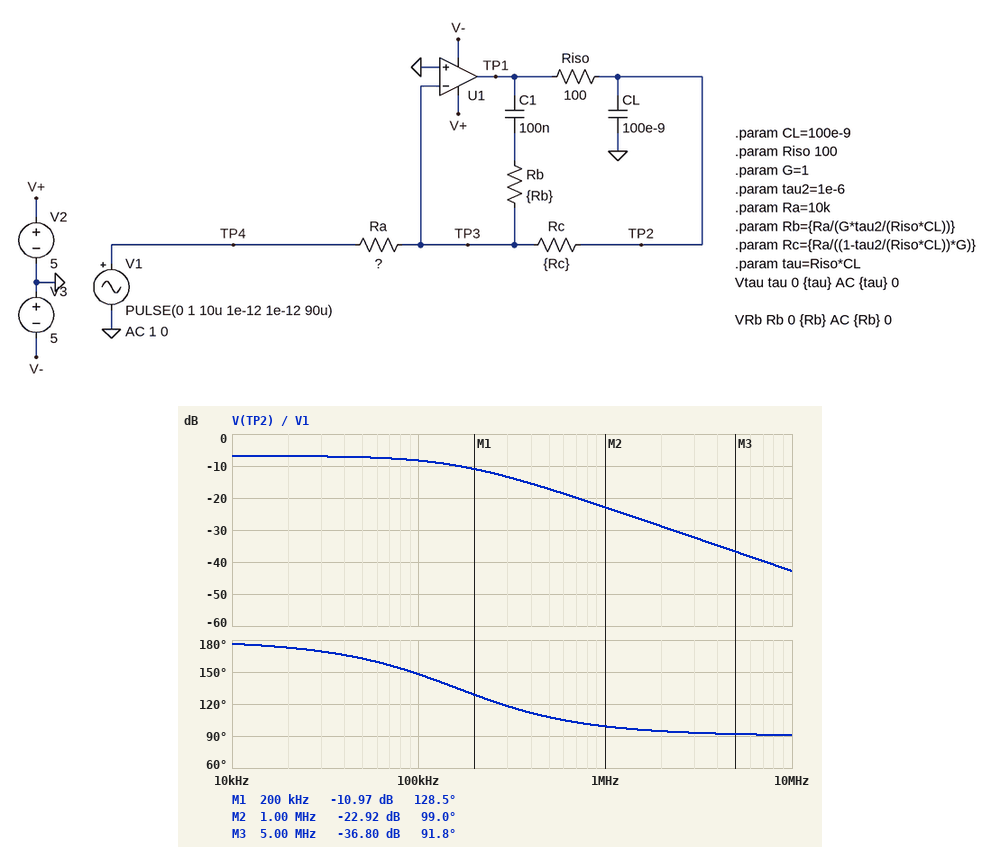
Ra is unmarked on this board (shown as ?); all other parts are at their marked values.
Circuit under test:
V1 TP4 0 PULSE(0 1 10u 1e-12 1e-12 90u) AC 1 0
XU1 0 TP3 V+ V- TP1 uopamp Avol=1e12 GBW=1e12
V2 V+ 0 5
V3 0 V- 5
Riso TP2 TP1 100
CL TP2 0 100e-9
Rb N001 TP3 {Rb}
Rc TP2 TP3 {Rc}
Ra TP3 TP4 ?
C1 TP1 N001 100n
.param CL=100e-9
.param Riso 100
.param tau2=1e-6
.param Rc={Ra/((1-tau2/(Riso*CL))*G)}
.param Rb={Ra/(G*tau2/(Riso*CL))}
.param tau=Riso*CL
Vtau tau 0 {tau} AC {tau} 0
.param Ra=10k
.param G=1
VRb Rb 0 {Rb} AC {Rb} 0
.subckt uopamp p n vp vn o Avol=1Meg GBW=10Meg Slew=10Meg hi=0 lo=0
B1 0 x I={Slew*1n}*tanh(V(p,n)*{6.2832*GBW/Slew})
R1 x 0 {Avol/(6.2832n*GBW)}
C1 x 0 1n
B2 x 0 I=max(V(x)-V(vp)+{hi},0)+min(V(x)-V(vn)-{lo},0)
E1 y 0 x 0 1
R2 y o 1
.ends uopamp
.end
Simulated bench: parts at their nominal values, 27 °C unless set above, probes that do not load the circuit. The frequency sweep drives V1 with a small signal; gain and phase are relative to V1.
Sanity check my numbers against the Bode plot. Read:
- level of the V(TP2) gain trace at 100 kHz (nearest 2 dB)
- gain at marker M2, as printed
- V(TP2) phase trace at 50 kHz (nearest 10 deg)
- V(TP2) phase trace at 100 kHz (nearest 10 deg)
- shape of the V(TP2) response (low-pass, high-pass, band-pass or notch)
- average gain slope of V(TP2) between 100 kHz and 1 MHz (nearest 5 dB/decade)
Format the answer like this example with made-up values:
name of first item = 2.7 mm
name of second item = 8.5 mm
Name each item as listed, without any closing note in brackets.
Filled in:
level of the V(TP2) gain trace at 100 kHz = -8 dB
gain at marker M2, as printed = -22.92 dB
V(TP2) phase trace at 50 kHz = 160 deg
V(TP2) phase trace at 100 kHz = 150 deg
shape of the V(TP2) response = low-pass
average gain slope of V(TP2) between 100 kHz and 1 MHz = -15 dB/decade
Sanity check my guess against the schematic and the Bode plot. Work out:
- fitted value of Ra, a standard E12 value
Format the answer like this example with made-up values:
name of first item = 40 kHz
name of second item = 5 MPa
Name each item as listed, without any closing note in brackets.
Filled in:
fitted value of Ra, a standard E12 value = 22 kΩ
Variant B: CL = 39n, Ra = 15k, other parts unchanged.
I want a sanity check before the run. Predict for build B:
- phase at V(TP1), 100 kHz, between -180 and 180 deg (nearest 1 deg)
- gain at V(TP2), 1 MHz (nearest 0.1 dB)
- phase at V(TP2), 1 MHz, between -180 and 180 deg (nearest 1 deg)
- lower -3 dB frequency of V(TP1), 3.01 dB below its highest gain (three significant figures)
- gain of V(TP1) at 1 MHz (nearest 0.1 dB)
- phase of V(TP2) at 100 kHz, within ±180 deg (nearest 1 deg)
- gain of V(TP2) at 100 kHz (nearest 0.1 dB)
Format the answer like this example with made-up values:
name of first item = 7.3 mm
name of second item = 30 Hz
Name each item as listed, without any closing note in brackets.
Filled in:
phase at V(TP1), 100 kHz, between -180 and 180 deg = -126 deg
gain at V(TP2), 1 MHz = -12.0 dB
phase at V(TP2), 1 MHz, between -180 and 180 deg = 112 deg
lower -3 dB frequency of V(TP1), 3.01 dB below its highest gain = 404 kHz
gain of V(TP1) at 1 MHz = 15.8 dB
phase of V(TP2) at 100 kHz, within ±180 deg = 166 deg
gain of V(TP2) at 100 kHz = -3.8 dB
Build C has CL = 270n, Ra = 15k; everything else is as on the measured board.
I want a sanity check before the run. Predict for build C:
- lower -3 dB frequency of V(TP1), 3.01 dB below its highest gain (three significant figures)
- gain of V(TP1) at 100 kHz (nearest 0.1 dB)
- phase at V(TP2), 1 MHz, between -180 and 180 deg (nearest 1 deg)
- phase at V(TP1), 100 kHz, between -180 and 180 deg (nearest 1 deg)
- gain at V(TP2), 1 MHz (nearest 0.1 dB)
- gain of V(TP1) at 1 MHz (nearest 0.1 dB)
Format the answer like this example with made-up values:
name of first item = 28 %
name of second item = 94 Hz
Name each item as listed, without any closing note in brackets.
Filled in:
lower -3 dB frequency of V(TP1), 3.01 dB below its highest gain = 58.4 kHz
gain of V(TP1) at 100 kHz = 15.2 dB
phase at V(TP2), 1 MHz, between -180 and 180 deg = 93 deg
phase at V(TP1), 100 kHz, between -180 and 180 deg = -153 deg
gain at V(TP2), 1 MHz = -28.1 dB
gain of V(TP1) at 1 MHz = 16.5 dB
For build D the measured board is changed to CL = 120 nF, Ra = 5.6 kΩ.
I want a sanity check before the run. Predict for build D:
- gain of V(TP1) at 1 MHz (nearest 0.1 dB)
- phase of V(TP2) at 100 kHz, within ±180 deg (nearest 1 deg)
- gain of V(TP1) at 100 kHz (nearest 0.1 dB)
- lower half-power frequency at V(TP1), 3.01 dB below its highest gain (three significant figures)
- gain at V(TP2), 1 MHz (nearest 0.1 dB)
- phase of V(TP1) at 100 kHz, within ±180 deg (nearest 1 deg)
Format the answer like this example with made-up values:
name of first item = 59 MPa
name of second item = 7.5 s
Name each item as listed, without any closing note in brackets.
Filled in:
gain of V(TP1) at 1 MHz = 25.0 dB
phase of V(TP2) at 100 kHz, within ±180 deg = 143 deg
gain of V(TP1) at 100 kHz = 20.7 dB
lower half-power frequency at V(TP1), 3.01 dB below its highest gain = 131 kHz
gain at V(TP2), 1 MHz = -12.6 dB
phase of V(TP1) at 100 kHz, within ±180 deg = -135 deg
